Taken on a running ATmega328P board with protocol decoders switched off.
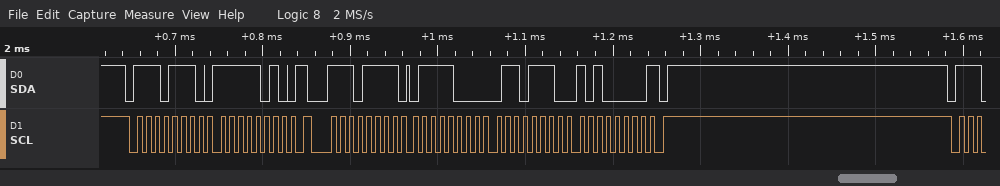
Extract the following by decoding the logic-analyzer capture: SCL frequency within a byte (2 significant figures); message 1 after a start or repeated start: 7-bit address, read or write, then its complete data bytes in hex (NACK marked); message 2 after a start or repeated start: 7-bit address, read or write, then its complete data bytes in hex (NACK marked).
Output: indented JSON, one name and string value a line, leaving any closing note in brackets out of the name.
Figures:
{
  "SCL frequency within a byte": "100 kHz",
  "message 1 after a start or repeated start: 7-bit address, read or write, then its complete data bytes in hex": "0x77 write: FA",
  "message 2 after a start or repeated start: 7-bit address, read or write, then its complete data bytes in hex": "0x77 read: 78 6E A0 NACK"
}
